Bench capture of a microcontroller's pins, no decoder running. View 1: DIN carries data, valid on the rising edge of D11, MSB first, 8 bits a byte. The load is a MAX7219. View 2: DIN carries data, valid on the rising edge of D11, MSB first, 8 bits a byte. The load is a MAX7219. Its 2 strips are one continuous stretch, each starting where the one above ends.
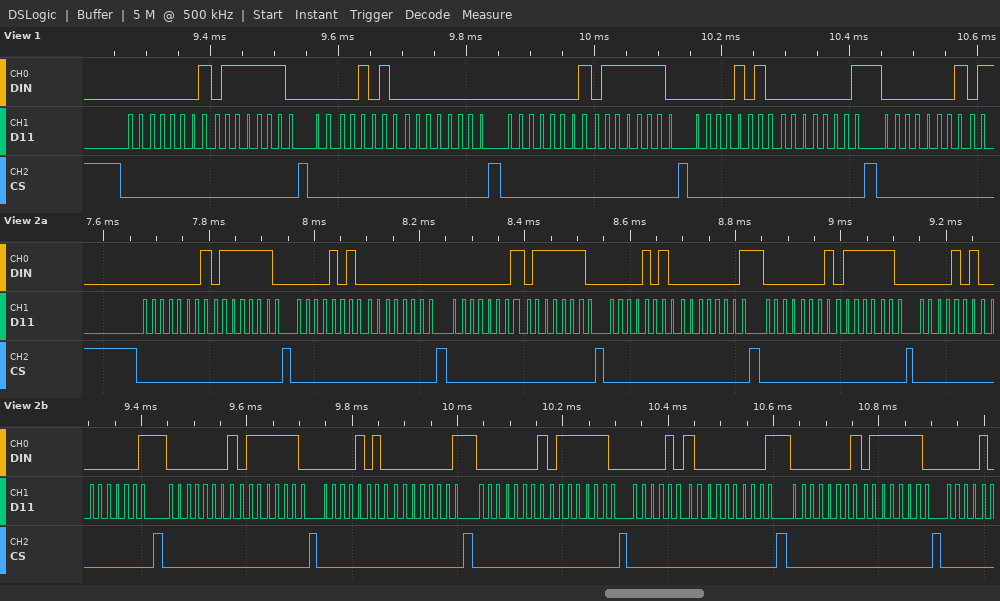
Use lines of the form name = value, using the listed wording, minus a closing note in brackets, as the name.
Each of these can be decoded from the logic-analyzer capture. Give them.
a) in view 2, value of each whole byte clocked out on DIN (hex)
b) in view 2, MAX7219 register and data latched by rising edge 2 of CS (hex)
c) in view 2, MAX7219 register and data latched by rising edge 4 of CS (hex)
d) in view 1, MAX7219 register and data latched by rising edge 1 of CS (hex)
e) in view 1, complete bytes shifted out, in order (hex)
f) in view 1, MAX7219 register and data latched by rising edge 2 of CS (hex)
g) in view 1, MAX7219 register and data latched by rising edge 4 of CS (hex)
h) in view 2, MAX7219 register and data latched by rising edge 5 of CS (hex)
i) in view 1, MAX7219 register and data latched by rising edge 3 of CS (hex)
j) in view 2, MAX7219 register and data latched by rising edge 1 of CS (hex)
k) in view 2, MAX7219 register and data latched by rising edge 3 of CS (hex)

in view 2, value of each whole byte clocked out on DIN = 01 7E 0A 00 01 7E 0A 01 01 7E 0A 01 01 7E 0A 01 01 7E 0A 01 01 7E
in view 2, MAX7219 register and data latched by rising edge 2 of CS = register 0xA, data 0x00
in view 2, MAX7219 register and data latched by rising edge 4 of CS = register 0xA, data 0x01
in view 1, MAX7219 register and data latched by rising edge 1 of CS = register 0x1, data 0x7E
in view 1, complete bytes shifted out, in order = 0x01 0x7E 0x0A 0x00 0x01 0x7E 0x0A 0x01 0x01
in view 1, MAX7219 register and data latched by rising edge 2 of CS = register 0xA, data 0x00
in view 1, MAX7219 register and data latched by rising edge 4 of CS = register 0xA, data 0x01
in view 2, MAX7219 register and data latched by rising edge 5 of CS = register 0x1, data 0x7E
in view 1, MAX7219 register and data latched by rising edge 3 of CS = register 0x1, data 0x7E
in view 2, MAX7219 register and data latched by rising edge 1 of CS = register 0x1, data 0x7E
in view 2, MAX7219 register and data latched by rising edge 3 of CS = register 0x1, data 0x7E
